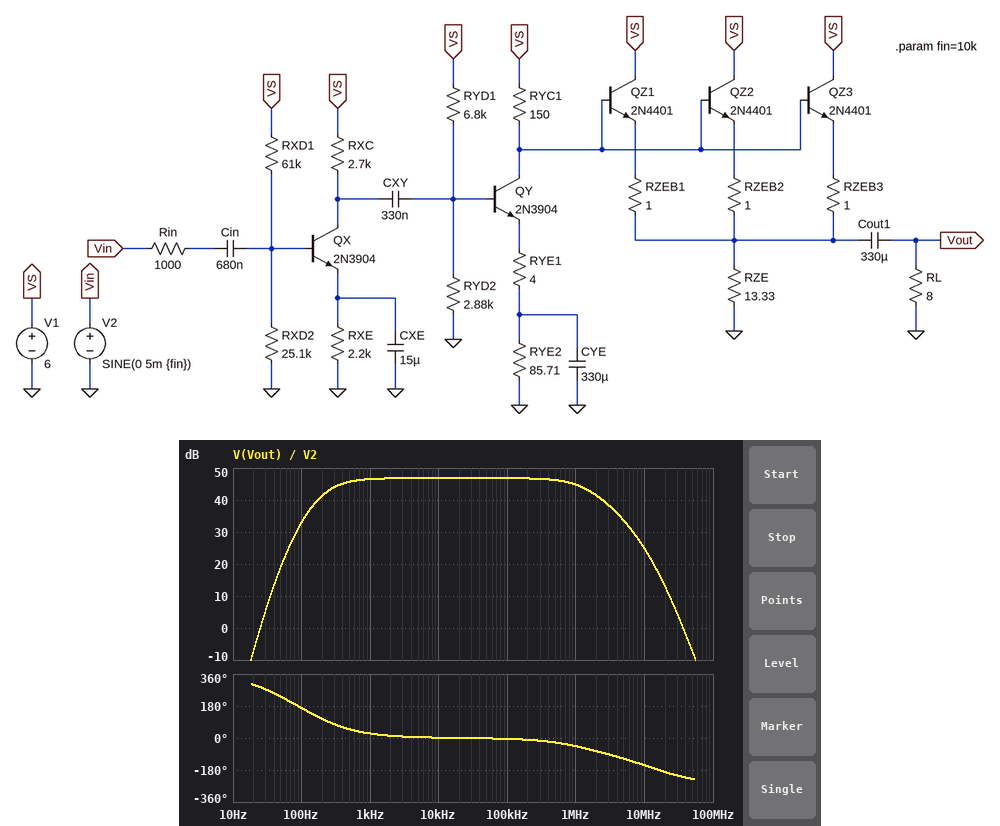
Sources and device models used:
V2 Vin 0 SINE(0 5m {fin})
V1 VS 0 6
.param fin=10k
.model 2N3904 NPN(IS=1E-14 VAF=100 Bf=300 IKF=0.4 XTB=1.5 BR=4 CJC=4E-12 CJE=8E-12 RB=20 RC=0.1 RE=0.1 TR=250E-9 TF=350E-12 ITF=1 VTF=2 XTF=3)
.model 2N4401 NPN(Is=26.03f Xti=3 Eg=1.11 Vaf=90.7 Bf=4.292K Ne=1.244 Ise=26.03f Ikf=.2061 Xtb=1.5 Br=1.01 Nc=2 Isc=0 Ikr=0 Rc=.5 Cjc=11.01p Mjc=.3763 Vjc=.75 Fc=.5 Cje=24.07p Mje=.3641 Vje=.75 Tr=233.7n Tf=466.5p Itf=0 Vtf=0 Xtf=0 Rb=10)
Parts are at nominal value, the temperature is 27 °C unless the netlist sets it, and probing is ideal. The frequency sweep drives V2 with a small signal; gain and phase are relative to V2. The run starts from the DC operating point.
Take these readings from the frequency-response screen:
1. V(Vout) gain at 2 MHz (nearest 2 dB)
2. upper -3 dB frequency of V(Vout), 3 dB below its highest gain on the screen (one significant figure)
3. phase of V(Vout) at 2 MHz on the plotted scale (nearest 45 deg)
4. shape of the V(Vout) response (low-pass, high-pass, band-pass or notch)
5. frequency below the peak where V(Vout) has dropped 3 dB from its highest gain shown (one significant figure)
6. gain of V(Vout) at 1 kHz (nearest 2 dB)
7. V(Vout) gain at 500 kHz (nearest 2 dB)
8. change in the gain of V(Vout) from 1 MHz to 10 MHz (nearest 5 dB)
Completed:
42 dB
1 MHz
-90 deg
band-pass
300 Hz
46 dB
46 dB
-20 dB
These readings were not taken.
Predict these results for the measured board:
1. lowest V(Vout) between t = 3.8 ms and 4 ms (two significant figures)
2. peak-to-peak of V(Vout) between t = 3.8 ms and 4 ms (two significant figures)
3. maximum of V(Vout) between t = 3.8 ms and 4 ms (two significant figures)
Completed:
-1.0 V
2.0 V
1.0 V
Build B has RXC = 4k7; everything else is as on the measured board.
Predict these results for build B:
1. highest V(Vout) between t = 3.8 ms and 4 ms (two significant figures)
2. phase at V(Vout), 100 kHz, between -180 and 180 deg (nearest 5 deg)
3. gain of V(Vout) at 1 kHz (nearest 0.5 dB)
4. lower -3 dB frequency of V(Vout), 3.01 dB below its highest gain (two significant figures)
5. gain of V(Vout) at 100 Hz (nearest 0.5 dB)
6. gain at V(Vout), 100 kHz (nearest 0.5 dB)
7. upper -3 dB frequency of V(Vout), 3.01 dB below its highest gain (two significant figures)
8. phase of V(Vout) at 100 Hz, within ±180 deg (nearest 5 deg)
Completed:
1.1 V
-5 deg
47.5 dB
260 Hz
36.0 dB
48.0 dB
1.1 MHz
155 deg
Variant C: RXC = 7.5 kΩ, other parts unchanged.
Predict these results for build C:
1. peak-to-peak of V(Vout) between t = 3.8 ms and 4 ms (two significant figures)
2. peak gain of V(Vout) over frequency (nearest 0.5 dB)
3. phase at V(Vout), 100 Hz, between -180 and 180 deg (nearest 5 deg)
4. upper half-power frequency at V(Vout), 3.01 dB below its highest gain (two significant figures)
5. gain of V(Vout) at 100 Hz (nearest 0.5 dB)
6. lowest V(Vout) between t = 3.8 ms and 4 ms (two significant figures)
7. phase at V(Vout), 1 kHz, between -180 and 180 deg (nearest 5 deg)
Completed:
2.4 V
48.5 dB
145 deg
990 kHz
38.0 dB
-1.2 V
20 deg
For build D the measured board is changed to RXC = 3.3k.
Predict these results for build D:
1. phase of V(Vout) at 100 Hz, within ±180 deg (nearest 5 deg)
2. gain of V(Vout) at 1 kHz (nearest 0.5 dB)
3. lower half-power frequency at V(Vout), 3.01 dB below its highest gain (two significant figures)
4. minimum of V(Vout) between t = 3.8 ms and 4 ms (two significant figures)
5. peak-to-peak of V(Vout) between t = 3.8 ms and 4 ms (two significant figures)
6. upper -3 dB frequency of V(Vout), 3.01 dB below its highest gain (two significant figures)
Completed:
165 deg
47.0 dB
280 Hz
-1.1 V
2.1 V
1.2 MHz
